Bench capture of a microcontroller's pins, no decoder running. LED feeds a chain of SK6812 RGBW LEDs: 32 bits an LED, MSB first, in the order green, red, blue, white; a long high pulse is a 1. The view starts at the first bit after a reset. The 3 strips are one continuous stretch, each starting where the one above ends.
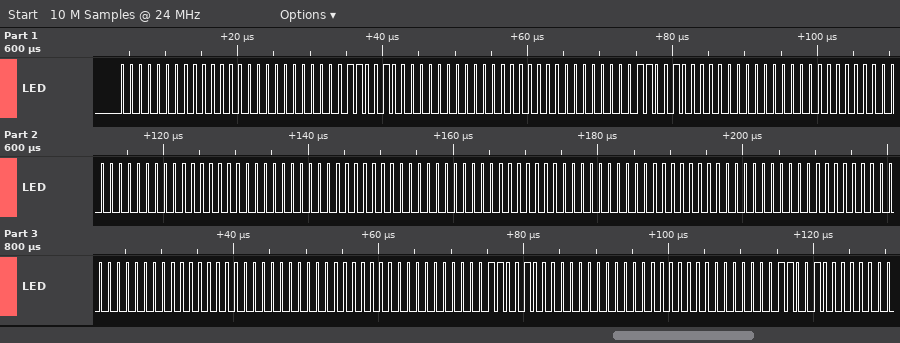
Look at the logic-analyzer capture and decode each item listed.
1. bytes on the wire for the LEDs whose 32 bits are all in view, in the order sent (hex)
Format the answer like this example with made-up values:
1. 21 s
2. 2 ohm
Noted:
1. 00 00 00 64 00 00 00 64 00 00 00 00 00 00 00 00 00 00 00 00 00 00 00 00 00 00 00 64 00 00 00 64
